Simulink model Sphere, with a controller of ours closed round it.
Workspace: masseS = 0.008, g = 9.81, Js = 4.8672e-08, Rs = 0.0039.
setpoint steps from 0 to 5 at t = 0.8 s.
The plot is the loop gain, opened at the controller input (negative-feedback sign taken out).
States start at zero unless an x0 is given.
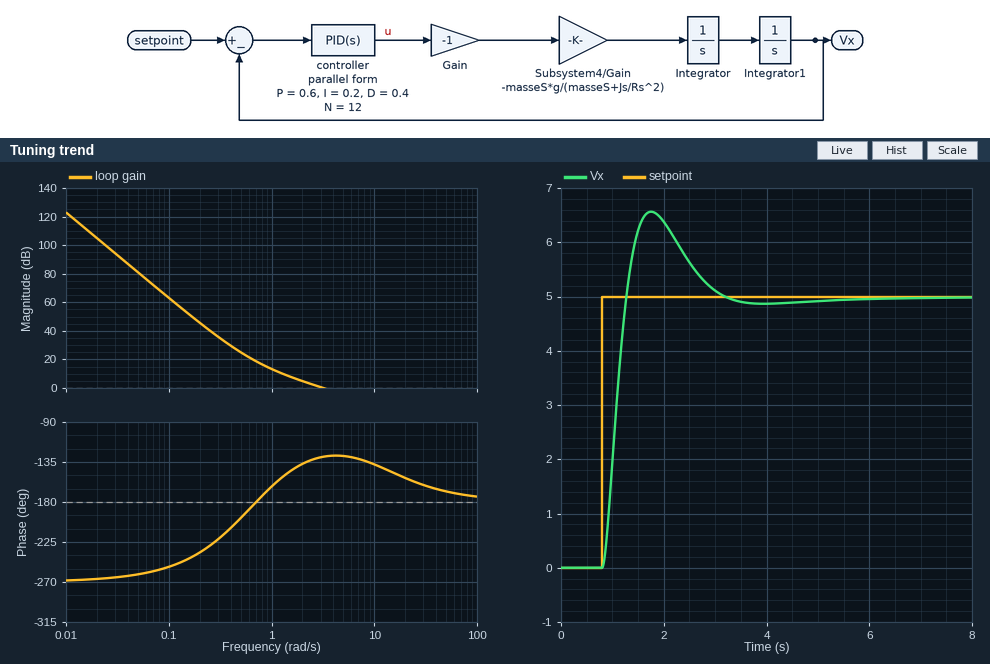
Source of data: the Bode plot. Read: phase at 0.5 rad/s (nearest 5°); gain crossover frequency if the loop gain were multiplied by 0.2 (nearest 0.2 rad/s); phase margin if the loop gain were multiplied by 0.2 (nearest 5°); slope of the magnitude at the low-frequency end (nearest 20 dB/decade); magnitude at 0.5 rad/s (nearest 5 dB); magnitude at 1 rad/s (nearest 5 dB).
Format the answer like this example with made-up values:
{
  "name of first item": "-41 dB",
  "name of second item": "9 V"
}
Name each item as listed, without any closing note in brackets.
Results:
{
  "phase at 0.5 rad/s": "-200°",
  "gain crossover frequency if the loop gain were multiplied by 0.2": "1.0 rad/s",
  "phase margin if the loop gain were multiplied by 0.2": "15°",
  "slope of the magnitude at the low-frequency end": "-60 dB/decade",
  "magnitude at 0.5 rad/s": "25 dB",
  "magnitude at 1 rad/s": "15 dB"
}
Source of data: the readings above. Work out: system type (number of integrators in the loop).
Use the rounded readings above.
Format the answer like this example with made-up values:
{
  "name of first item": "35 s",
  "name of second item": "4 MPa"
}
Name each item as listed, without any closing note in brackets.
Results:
{
  "system type": "3"
}
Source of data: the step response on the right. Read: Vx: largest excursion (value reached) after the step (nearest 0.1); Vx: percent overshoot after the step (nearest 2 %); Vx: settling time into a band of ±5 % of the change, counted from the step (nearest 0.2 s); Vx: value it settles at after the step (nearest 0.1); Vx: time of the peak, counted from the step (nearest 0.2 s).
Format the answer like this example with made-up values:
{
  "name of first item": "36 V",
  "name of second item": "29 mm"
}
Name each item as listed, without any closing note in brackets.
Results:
{
  "Vx: largest excursion (value reached) after the step": "6.6",
  "Vx: percent overshoot after the step": "32 %",
  "Vx: settling time into a band of ±5 % of the change, counted from the step": "2.0 s",
  "Vx: value it settles at after the step": "5.0",
  "Vx: time of the peak, counted from the step": "1.0 s"
}
